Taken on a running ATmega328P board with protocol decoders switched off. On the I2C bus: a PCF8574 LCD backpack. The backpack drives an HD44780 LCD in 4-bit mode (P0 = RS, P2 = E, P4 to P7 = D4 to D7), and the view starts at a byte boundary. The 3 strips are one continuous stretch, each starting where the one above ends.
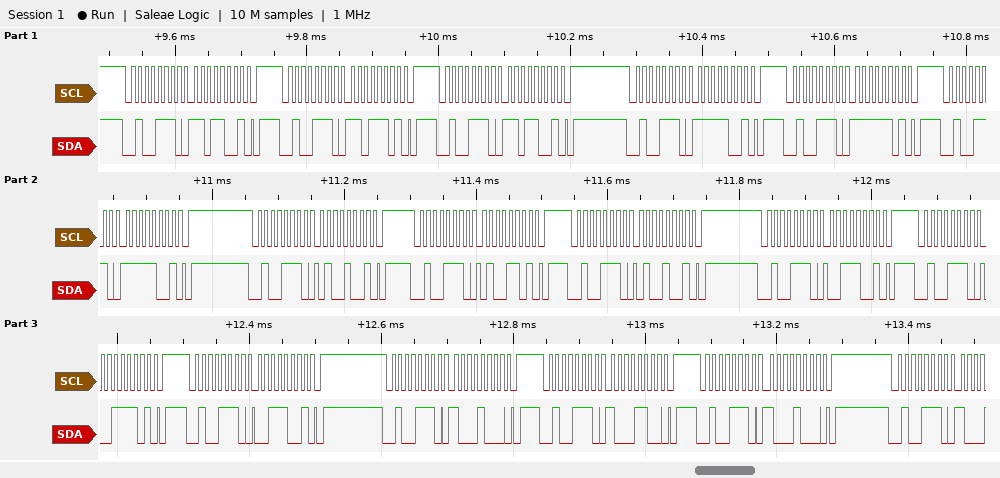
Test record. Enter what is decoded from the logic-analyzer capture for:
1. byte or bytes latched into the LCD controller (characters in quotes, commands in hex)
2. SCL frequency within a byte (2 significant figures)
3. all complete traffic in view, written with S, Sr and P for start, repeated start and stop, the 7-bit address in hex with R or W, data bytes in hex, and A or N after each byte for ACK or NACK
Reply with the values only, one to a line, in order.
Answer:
data 0xDF 'C'
100 kHz
S 27W A D9 A P S 27W A DD A P S 27W A D9 A P S 27W A F9 A P S 27W A FD A P S 27W A F9 A P S 27W A 49 A P S 27W A 4D A P S 27W A 49 A P S 27W A 39 A P S 27W A 3D A P S 27W A 39 A P S 27W A 88 A P S 27W A 8C A P S 27W A 88 A P S 27W A
